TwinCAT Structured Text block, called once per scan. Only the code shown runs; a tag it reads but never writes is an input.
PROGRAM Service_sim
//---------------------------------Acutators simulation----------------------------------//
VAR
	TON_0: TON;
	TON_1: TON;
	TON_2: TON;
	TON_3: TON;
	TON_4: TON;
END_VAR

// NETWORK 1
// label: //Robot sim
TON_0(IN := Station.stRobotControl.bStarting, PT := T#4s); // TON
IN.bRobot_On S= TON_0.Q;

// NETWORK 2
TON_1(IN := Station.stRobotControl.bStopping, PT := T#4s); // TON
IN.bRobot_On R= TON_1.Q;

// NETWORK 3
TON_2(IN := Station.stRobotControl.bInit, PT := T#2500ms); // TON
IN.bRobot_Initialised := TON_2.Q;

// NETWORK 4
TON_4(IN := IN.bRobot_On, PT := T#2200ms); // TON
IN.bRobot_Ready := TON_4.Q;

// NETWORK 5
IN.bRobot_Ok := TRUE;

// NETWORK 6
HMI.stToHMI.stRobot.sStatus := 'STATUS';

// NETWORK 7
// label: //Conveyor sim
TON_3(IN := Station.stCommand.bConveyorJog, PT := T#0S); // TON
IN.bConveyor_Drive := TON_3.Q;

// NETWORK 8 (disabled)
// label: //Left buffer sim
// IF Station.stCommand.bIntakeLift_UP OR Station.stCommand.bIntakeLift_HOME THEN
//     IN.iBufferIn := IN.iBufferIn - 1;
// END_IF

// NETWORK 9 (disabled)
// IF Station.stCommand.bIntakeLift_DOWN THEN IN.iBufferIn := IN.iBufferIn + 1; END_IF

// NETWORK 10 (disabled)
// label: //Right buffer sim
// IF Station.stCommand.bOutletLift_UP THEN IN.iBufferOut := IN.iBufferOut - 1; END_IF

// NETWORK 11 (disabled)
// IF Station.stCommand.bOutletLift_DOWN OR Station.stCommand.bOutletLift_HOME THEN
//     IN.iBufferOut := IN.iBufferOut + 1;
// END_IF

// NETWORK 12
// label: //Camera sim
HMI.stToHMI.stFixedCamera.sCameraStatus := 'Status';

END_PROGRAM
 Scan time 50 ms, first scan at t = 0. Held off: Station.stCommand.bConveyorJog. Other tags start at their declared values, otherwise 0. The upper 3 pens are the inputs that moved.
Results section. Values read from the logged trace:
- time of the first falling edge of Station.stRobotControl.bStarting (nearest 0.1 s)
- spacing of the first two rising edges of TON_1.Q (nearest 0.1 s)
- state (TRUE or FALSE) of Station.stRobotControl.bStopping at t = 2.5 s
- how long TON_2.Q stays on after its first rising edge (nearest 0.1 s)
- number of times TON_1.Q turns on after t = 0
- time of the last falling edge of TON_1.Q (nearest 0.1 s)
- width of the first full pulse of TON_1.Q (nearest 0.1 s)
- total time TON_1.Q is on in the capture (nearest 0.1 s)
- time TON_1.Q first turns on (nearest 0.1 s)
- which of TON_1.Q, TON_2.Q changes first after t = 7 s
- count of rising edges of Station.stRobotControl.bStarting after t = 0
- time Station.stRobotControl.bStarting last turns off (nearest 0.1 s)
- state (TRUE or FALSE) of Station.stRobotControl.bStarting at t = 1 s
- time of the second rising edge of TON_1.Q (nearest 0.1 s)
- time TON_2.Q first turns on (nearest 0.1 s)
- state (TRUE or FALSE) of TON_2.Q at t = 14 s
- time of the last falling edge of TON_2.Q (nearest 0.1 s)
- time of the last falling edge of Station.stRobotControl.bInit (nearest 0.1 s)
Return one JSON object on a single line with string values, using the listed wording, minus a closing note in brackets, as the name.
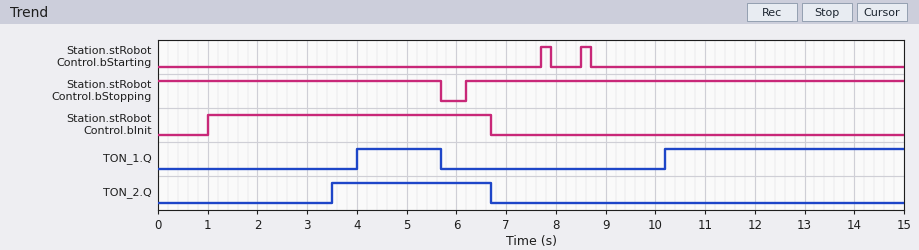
{"time of the first falling edge of Station.stRobotControl.bStarting": "7.9 s", "spacing of the first two rising edges of TON_1.Q": "6.2 s", "state (TRUE or FALSE) of Station.stRobotControl.bStopping at t = 2.5 s": "TRUE", "how long TON_2.Q stays on after its first rising edge": "3.2 s", "number of times TON_1.Q turns on after t = 0": "2", "time of the last falling edge of TON_1.Q": "5.7 s", "width of the first full pulse of TON_1.Q": "1.7 s", "total time TON_1.Q is on in the capture": "6.5 s", "time TON_1.Q first turns on": "4.0 s", "which of TON_1.Q, TON_2.Q changes first after t = 7 s": "TON_1.Q", "count of rising edges of Station.stRobotControl.bStarting after t = 0": "2", "time Station.stRobotControl.bStarting last turns off": "8.7 s", "state (TRUE or FALSE) of Station.stRobotControl.bStarting at t = 1 s": "FALSE", "time of the second rising edge of TON_1.Q": "10.2 s", "time TON_2.Q first turns on": "3.5 s", "state (TRUE or FALSE) of TON_2.Q at t = 14 s": "FALSE", "time of the last falling edge of TON_2.Q": "6.7 s", "time of the last falling edge of Station.stRobotControl.bInit": "6.7 s"}
